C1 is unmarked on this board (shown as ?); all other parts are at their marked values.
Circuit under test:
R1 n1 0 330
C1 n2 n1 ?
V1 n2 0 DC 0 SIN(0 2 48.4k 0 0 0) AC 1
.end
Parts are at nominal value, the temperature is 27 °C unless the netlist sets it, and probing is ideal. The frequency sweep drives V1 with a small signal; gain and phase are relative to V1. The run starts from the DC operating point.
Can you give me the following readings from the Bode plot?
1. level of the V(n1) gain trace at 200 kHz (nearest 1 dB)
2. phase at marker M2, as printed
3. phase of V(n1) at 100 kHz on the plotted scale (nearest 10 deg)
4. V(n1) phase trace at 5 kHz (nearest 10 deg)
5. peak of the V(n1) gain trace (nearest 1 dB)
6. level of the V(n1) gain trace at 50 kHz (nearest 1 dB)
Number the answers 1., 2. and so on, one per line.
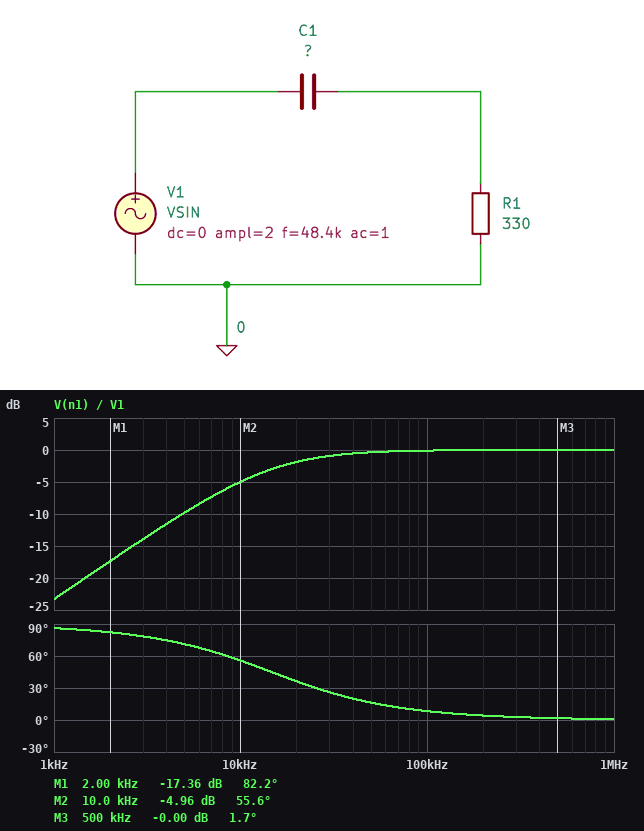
1. 0 dB
2. 55.6 deg
3. 10 deg
4. 70 deg
5. 0 dB
6. 0 dB
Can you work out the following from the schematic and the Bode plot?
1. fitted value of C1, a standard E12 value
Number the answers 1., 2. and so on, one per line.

1. 33 nF
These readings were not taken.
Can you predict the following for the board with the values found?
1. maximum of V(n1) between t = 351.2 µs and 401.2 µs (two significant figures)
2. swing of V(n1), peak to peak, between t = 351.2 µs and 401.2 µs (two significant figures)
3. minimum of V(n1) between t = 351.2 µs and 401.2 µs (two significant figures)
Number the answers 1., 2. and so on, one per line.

1. 1.9 V
2. 3.8 V
3. -1.9 V
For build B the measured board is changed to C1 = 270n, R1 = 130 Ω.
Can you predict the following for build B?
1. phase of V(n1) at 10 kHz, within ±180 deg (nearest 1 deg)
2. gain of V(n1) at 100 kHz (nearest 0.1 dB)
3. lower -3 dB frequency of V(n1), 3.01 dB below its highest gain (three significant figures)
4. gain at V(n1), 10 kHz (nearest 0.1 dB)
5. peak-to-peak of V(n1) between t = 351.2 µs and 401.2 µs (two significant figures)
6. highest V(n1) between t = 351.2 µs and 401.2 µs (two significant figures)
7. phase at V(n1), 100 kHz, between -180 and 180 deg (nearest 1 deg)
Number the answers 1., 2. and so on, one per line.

1. 24 deg
2. 0 dB
3. 4.53 kHz
4. -0.8 dB
5. 4.0 V
6. 2.0 V
7. 3 deg
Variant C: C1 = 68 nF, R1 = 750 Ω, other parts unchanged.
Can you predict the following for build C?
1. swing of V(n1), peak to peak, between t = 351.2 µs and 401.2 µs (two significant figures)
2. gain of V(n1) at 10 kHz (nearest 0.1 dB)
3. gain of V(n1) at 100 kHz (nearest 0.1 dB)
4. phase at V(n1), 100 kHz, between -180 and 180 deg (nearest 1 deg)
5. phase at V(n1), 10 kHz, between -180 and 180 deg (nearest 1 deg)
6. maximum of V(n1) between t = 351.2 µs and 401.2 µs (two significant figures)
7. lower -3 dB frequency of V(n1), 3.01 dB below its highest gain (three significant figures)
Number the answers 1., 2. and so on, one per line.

1. 4.0 V
2. -0.4 dB
3. 0 dB
4. 2 deg
5. 17 deg
6. 2.0 V
7. 3.12 kHz
